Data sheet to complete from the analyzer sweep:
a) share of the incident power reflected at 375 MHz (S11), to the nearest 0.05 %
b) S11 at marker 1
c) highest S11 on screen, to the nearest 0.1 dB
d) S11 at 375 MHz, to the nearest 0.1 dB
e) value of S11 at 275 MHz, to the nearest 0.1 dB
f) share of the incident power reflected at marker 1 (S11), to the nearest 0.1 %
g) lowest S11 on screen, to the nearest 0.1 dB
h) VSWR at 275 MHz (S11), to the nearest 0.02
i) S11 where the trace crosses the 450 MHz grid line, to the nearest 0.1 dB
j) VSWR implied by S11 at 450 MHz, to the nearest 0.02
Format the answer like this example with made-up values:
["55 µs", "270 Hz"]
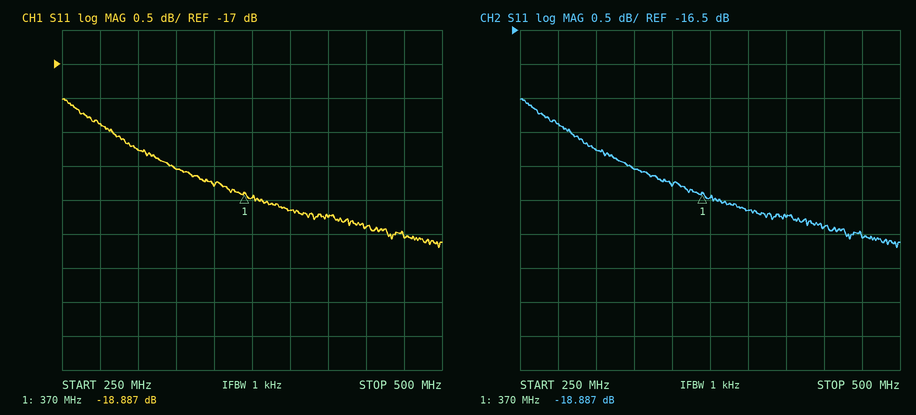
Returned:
["1.25 %", "-18.887 dB", "-17.5 dB", "-19.0 dB", "-17.9 dB", "1.3 %", "-19.7 dB", "1.30", "-19.4 dB", "1.24"]
